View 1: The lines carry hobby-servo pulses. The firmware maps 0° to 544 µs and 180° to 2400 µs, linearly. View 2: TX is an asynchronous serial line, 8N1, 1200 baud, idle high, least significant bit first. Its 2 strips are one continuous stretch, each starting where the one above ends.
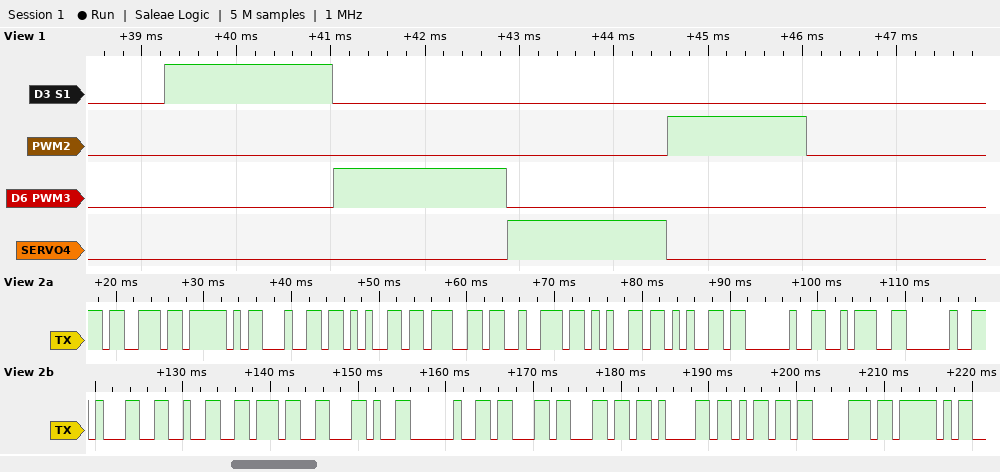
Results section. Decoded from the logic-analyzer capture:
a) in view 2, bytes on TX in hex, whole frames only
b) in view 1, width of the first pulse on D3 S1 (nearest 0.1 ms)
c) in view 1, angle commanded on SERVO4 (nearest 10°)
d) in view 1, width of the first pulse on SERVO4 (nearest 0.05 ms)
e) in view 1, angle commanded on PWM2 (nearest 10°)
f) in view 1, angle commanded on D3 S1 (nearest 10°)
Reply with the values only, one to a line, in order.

73 5F 64 65 67 72 65 65 20 3A 20 31 32 37 2C 20 63 6C 61 6D 70 5F
1.8 ms
110°
1.70 ms
90°
120°
